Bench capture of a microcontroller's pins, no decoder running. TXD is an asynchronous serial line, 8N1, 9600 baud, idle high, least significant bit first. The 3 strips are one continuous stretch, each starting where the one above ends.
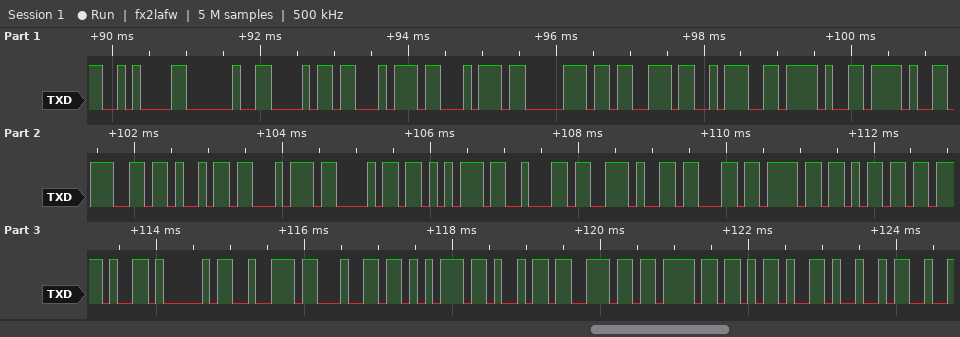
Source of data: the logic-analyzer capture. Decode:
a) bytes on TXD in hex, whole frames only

0A 20 68 74 74 70 73 3A 2F 2F 67 69 74 68 75 62 2E 63 6F 6D 2F 41 72 64 75 69 6E 6F 2D 49
